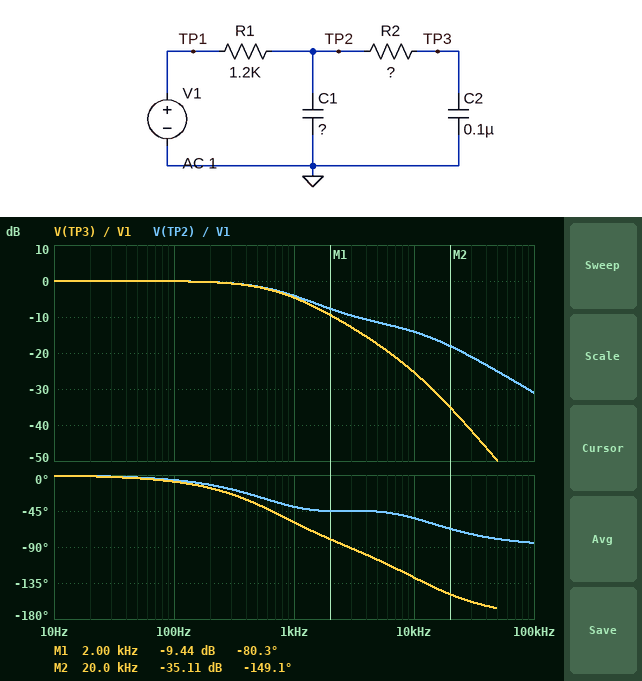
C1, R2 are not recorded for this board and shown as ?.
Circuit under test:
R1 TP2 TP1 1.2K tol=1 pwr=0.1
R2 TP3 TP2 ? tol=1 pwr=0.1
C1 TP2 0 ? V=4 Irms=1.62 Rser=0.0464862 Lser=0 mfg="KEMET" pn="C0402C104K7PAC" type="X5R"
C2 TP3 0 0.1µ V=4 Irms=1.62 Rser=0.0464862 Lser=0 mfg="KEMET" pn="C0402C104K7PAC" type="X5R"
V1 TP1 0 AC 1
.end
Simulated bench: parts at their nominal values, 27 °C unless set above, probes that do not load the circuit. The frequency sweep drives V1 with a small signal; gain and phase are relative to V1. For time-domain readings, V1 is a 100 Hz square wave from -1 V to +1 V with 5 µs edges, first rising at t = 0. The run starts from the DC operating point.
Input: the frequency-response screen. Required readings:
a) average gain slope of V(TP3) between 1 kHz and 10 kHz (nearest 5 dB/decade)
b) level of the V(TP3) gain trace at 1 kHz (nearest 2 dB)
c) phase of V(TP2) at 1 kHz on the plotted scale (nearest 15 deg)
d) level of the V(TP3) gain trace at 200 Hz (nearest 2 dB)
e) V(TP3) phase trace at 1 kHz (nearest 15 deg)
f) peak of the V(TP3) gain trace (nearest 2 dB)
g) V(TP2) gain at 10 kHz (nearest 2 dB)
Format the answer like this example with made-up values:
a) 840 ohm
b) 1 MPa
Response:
a) -20 dB/decade
b) -4 dB
c) -45 deg
d) 0 dB
e) -60 deg
f) 0 dB
g) -14 dB
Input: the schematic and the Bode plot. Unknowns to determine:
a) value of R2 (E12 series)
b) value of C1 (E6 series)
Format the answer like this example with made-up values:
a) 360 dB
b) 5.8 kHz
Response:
a) 560 Ω
b) 47 nF
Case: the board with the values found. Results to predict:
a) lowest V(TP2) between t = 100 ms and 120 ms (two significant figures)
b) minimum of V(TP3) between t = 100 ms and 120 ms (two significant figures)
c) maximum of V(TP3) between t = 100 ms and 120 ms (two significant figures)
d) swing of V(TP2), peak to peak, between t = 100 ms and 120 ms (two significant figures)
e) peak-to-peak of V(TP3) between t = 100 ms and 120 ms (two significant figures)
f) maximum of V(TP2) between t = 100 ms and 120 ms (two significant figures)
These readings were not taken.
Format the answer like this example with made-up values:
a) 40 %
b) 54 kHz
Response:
a) -1.0 V
b) -1.0 V
c) 1.0 V
d) 2.0 V
e) 2.0 V
f) 1.0 V
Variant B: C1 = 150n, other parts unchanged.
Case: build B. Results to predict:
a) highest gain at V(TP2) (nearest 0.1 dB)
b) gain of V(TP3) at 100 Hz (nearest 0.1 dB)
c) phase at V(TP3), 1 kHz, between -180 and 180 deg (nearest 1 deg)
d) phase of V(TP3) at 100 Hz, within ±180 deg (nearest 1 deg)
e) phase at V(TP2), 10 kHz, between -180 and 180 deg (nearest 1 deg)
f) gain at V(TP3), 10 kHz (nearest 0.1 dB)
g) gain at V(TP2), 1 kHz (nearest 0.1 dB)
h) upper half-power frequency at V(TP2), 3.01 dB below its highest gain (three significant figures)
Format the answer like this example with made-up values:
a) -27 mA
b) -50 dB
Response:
a) 0 dB
b) -0.2 dB
c) -75 deg
d) -13 deg
e) -76 deg
f) -33.0 dB
g) -6.8 dB
h) 500 Hz
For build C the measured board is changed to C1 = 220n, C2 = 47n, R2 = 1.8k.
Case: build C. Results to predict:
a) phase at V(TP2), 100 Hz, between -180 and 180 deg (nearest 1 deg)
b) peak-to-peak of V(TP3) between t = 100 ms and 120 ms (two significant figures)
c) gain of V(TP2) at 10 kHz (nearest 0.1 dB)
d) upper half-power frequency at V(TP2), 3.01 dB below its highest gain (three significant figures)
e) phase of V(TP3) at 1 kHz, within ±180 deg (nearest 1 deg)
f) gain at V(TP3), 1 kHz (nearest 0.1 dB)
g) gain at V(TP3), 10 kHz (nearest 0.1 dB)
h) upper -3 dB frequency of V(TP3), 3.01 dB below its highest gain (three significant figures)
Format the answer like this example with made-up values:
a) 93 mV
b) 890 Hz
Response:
a) -11 deg
b) 2.0 V
c) -24.5 dB
d) 481 Hz
e) -87 deg
f) -8.1 dB
g) -39.2 dB
h) 453 Hz
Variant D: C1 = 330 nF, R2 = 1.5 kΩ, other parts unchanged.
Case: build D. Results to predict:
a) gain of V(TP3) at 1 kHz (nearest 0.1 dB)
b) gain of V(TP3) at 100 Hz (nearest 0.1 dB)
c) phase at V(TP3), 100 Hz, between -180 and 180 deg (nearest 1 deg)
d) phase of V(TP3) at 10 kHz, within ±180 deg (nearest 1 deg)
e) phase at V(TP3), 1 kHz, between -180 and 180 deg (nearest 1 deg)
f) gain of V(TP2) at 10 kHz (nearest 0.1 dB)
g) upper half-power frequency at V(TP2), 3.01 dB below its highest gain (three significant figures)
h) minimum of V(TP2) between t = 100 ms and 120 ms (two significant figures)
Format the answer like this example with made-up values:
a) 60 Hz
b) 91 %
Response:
a) -12.9 dB
b) -0.5 dB
c) -23 deg
d) -170 deg
e) -108 deg
f) -28.0 dB
g) 295 Hz
h) -1.0 V
